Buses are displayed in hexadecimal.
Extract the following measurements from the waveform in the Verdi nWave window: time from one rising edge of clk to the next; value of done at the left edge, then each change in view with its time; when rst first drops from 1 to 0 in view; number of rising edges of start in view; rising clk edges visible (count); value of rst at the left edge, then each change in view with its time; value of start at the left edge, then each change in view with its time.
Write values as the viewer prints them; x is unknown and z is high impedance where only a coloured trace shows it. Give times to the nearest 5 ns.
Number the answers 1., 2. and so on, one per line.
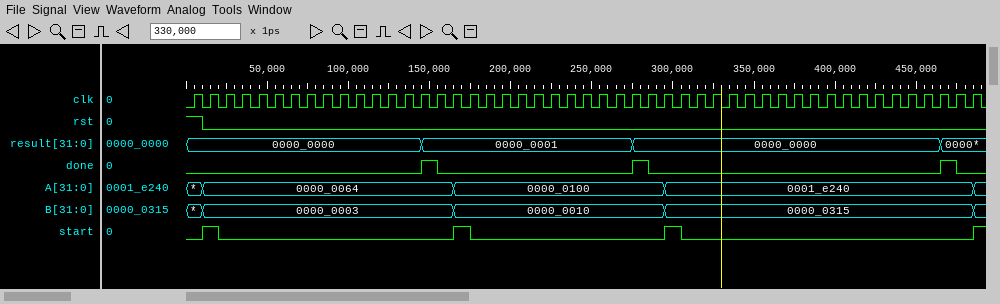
1. 10 ns
2. 0, 1 at 145 ns, 0 at 155 ns, 1 at 275 ns, 0 at 285 ns, 1 at 465 ns, 0 at 475 ns
3. 10 ns
4. 4
5. 49
6. 1, 0 at 10 ns
7. 0, 1 at 10 ns, 0 at 20 ns, 1 at 165 ns, 0 at 175 ns, 1 at 295 ns, 0 at 305 ns, 1 at 485 ns
